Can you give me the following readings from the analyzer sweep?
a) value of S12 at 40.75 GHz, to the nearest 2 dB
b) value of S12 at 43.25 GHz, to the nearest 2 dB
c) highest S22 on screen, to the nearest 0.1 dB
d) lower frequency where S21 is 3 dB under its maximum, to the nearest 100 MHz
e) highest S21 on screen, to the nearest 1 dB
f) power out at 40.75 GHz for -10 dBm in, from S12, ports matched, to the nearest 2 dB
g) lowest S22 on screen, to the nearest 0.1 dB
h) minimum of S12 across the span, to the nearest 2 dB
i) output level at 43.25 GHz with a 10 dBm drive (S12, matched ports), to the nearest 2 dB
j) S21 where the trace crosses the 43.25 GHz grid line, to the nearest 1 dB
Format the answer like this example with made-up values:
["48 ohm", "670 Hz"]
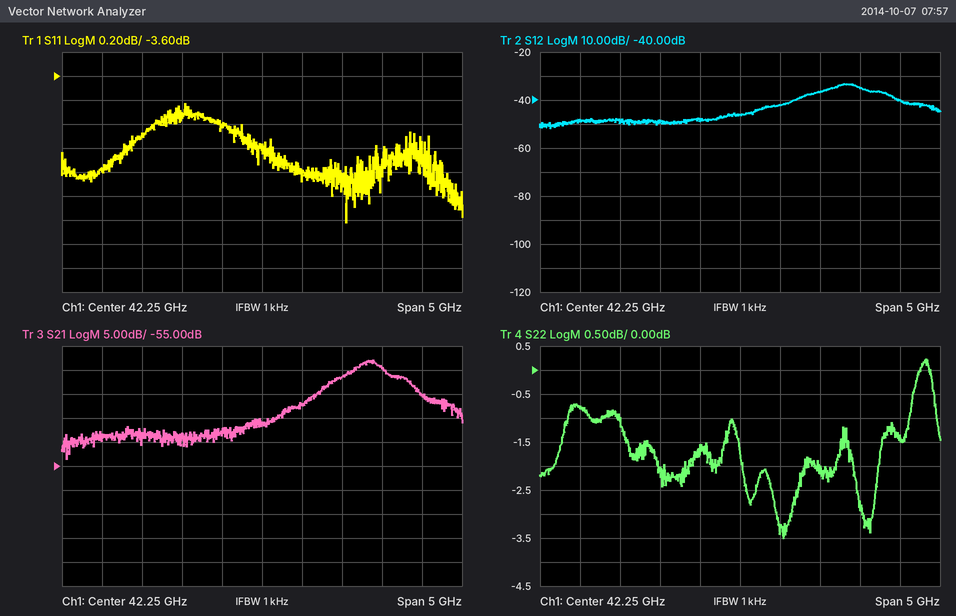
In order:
["-48 dB", "-36 dB", "0.2 dB", "43.3 GHz", "-33 dB", "-58 dBm", "-3.5 dB", "-52 dB", "-26 dBm", "-36 dB"]
